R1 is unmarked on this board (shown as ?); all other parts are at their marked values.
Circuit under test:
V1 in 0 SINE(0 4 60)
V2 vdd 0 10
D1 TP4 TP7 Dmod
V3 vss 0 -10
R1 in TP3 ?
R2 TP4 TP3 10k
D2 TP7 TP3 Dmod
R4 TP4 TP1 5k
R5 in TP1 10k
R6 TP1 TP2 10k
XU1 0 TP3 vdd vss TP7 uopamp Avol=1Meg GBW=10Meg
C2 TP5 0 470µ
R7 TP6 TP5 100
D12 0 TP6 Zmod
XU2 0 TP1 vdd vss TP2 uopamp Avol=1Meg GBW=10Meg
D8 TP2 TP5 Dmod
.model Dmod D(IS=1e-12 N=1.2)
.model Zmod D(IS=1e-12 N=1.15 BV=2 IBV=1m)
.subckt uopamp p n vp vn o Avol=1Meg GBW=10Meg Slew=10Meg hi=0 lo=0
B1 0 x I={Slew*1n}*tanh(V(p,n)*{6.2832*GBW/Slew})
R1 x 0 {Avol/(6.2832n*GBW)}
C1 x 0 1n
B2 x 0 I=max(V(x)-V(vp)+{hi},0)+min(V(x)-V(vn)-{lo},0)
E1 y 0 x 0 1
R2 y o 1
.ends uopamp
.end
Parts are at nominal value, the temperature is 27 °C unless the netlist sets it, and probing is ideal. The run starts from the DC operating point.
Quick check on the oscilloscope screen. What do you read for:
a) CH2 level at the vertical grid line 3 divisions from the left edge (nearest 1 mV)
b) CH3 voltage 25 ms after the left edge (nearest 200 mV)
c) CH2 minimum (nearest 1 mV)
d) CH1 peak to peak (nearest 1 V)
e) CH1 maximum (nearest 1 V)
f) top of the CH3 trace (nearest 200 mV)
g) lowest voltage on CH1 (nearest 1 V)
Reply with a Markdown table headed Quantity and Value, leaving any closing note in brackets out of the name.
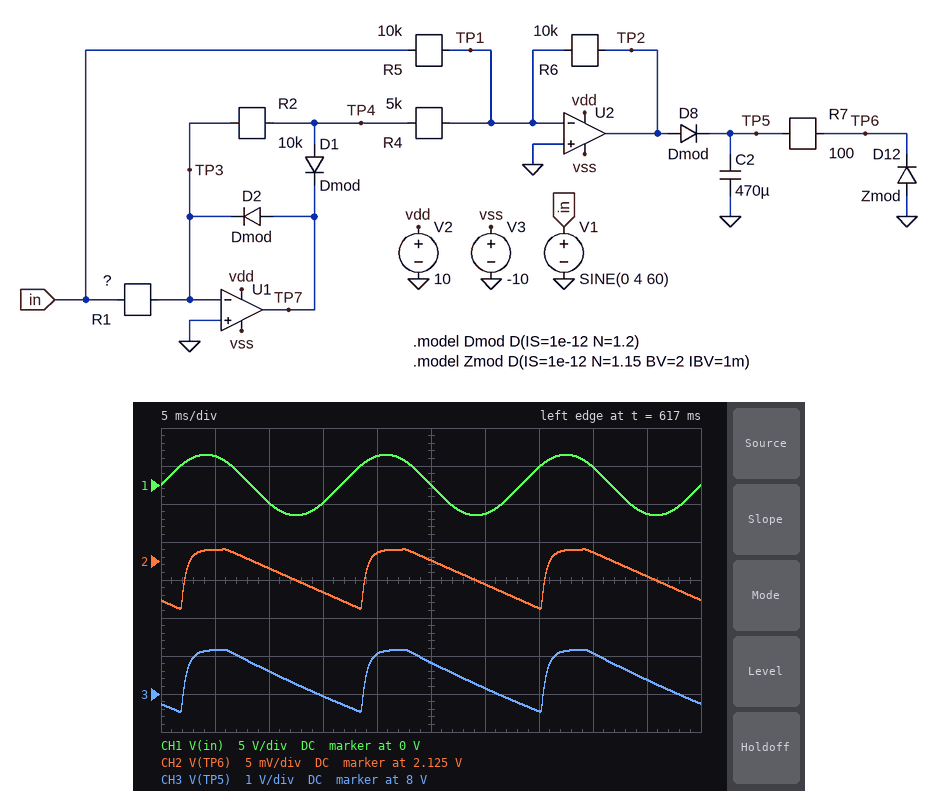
| Quantity | Value |
|---|---|
| CH2 level at the vertical grid line 3 divisions from the left edge | 2.121 V |
| CH3 voltage 25 ms after the left edge | 8.8 V |
| CH2 minimum | 2.119 V |
| CH1 peak to peak | 8 V |
| CH1 maximum | 4 V |
| top of the CH3 trace | 9.2 V |
| lowest voltage on CH1 | -4 V |
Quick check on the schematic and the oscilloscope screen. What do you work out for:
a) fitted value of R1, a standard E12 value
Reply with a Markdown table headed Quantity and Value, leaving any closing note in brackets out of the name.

| Quantity | Value |
|---|---|
| fitted value of R1, a standard E12 value | 4.7 kΩ |
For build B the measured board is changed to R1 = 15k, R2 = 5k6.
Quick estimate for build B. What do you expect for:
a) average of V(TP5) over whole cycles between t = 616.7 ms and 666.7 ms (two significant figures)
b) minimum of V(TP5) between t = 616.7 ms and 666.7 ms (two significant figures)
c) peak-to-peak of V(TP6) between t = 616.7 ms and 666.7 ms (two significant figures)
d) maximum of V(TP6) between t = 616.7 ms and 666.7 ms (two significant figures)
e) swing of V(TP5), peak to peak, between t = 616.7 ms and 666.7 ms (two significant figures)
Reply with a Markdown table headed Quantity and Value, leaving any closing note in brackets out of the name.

| Quantity | Value |
|---|---|
| average of V(TP5) over whole cycles between t = 616.7 ms and 666.7 ms | 3.1 V |
| minimum of V(TP5) between t = 616.7 ms and 666.7 ms | 2.9 V |
| peak-to-peak of V(TP6) between t = 616.7 ms and 666.7 ms | 9.2 mV |
| maximum of V(TP6) between t = 616.7 ms and 666.7 ms | 2.1 V |
| swing of V(TP5), peak to peak, between t = 616.7 ms and 666.7 ms | 320 mV |
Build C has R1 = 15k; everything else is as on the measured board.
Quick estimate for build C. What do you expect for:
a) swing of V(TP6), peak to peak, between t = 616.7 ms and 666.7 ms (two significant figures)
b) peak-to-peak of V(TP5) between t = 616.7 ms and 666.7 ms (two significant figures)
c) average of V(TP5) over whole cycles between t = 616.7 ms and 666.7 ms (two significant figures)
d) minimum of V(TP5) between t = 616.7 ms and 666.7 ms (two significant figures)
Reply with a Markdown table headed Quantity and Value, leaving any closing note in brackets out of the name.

| Quantity | Value |
|---|---|
| swing of V(TP6), peak to peak, between t = 616.7 ms and 666.7 ms | 9.2 mV |
| peak-to-peak of V(TP5) between t = 616.7 ms and 666.7 ms | 320 mV |
| average of V(TP5) over whole cycles between t = 616.7 ms and 666.7 ms | 3.1 V |
| minimum of V(TP5) between t = 616.7 ms and 666.7 ms | 2.9 V |
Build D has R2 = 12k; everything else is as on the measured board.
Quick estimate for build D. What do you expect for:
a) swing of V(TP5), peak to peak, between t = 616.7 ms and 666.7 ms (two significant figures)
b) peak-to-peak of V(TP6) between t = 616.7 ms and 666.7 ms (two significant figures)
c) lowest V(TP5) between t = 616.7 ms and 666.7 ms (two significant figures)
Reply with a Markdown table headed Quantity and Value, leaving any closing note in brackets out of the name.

| Quantity | Value |
|---|---|
| swing of V(TP5), peak to peak, between t = 616.7 ms and 666.7 ms | 1.5 V |
| peak-to-peak of V(TP6) between t = 616.7 ms and 666.7 ms | 7.2 mV |
| lowest V(TP5) between t = 616.7 ms and 666.7 ms | 7.6 V |
